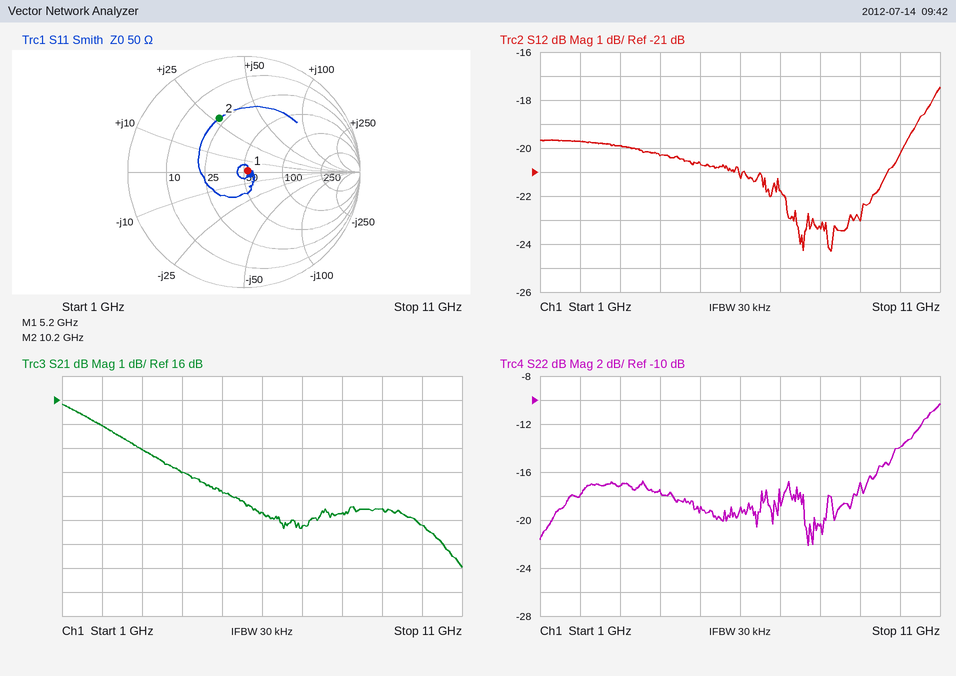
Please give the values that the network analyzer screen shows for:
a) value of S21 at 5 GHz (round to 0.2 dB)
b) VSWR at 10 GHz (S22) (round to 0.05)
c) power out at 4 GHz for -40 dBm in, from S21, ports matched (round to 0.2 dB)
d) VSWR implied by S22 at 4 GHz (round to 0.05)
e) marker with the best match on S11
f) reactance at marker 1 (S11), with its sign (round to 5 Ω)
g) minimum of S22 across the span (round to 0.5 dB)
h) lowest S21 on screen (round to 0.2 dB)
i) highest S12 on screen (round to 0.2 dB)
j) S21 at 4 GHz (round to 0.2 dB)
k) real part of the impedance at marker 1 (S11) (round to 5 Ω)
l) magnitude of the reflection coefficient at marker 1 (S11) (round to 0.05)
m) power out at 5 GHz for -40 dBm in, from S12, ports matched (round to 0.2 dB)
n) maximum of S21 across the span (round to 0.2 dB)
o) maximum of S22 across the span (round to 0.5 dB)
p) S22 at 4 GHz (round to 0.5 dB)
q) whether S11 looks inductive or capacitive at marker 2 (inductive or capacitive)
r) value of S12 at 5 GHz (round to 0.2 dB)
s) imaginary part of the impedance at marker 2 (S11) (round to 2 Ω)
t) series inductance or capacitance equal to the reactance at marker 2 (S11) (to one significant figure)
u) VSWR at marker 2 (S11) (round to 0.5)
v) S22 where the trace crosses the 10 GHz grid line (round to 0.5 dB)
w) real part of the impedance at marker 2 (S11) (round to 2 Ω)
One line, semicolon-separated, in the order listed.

12.2 dB; 1.50; -27.0 dBm; 1.30; marker 1; 0 Ω; -22.0 dB; 9.0 dB; -17.4 dB; 13.0 dB; 55 Ω; 0.05; -60.6 dBm; 15.8 dB; -10.5 dB; -17.5 dB; inductive; -20.6 dB; +28 Ω; 400 pH; 3.0; -14.0 dB; 22 Ω
